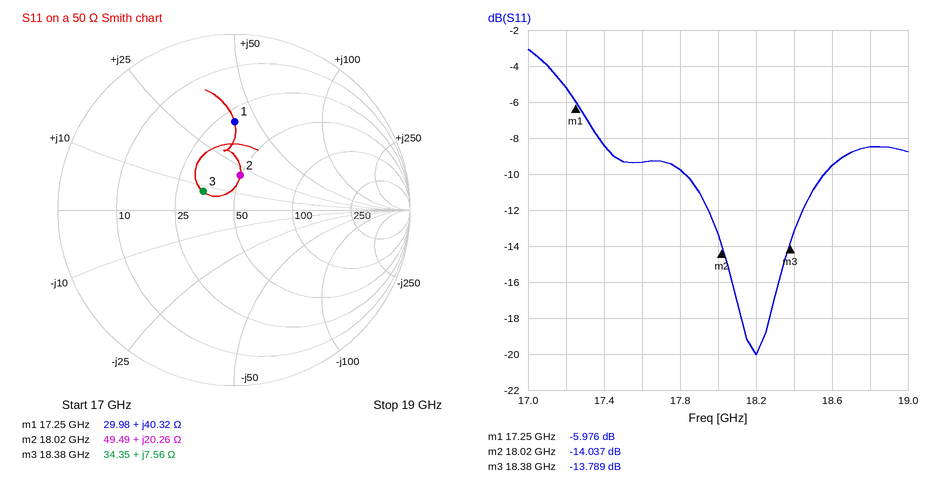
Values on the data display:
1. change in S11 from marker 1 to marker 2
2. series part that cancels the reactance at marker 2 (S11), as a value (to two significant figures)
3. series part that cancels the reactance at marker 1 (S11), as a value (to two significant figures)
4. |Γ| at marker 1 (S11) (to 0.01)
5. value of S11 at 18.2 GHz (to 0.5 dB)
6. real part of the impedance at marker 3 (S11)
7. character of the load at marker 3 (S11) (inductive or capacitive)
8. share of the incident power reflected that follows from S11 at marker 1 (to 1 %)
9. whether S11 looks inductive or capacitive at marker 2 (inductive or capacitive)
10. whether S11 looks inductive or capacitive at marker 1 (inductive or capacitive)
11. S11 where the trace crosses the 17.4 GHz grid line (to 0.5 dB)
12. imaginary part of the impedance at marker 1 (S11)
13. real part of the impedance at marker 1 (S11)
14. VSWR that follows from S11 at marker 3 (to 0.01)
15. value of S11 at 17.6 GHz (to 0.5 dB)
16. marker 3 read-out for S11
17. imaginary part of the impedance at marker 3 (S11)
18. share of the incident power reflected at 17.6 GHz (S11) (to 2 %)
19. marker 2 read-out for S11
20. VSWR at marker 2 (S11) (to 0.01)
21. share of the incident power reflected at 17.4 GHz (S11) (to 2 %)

-8.061 dB
440 fF
230 fF
0.50
-20.0 dB
34.35 Ω
inductive
25 %
inductive
inductive
-8.5 dB
+40.32 Ω
29.98 Ω
1.51
-9.5 dB
-13.789 dB
+7.56 Ω
12 %
-14.037 dB
1.50
14 %
